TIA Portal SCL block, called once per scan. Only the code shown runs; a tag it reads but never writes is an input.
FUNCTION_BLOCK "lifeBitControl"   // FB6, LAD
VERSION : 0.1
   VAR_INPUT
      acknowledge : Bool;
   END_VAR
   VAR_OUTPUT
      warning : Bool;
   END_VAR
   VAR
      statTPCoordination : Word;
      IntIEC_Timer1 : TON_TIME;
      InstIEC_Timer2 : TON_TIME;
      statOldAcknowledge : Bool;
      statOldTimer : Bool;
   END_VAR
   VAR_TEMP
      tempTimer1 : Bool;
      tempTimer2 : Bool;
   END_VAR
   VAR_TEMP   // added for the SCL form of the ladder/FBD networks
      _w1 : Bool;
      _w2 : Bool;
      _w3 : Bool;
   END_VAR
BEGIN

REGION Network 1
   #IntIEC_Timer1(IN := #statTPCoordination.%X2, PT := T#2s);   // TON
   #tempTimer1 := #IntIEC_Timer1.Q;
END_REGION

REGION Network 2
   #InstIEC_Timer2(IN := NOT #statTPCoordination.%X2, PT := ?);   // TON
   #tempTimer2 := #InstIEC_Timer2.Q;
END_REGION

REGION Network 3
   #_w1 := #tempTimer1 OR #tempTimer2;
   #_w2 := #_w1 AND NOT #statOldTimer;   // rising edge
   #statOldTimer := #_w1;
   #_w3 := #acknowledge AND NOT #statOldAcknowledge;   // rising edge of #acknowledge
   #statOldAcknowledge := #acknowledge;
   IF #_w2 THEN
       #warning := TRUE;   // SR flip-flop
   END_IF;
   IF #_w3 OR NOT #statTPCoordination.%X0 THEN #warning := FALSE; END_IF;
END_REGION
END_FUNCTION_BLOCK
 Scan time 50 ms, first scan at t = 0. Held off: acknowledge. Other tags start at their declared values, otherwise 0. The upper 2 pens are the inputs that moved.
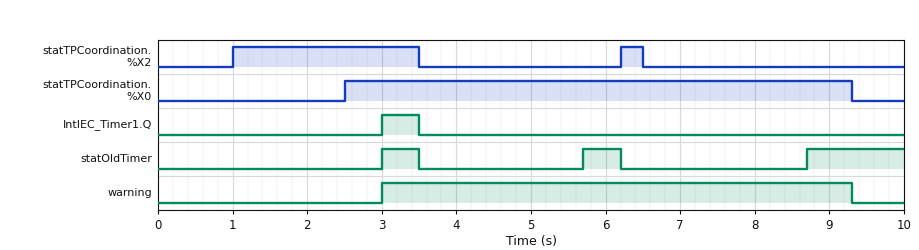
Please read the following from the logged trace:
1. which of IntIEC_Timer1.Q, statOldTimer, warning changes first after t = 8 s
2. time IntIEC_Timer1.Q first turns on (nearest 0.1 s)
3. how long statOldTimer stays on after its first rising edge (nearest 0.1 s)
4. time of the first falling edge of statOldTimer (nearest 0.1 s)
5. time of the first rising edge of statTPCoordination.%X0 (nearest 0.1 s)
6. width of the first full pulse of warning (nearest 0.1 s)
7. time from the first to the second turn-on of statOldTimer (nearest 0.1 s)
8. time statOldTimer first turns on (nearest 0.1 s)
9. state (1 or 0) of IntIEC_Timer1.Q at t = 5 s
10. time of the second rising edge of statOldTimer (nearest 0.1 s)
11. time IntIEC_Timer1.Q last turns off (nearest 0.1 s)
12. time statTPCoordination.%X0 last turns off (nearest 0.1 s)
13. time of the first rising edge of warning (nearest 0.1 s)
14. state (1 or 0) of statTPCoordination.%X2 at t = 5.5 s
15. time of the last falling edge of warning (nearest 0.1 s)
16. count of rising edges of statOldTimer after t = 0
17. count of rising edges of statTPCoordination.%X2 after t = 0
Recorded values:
statOldTimer
3.0 s
0.5 s
3.5 s
2.5 s
6.3 s
2.7 s
3.0 s
0
5.7 s
3.5 s
9.3 s
3.0 s
0
9.3 s
3
2
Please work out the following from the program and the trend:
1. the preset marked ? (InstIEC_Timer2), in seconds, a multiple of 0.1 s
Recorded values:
2.2 s
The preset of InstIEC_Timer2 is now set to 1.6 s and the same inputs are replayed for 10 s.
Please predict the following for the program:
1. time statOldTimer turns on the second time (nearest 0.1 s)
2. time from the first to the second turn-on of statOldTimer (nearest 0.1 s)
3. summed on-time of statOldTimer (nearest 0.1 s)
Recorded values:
5.1 s
2.1 s
3.5 s
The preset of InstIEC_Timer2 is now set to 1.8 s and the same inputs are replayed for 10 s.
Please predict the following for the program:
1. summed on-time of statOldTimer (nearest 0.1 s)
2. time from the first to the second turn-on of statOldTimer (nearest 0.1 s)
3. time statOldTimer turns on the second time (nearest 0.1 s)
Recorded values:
3.1 s
2.3 s
5.3 s
